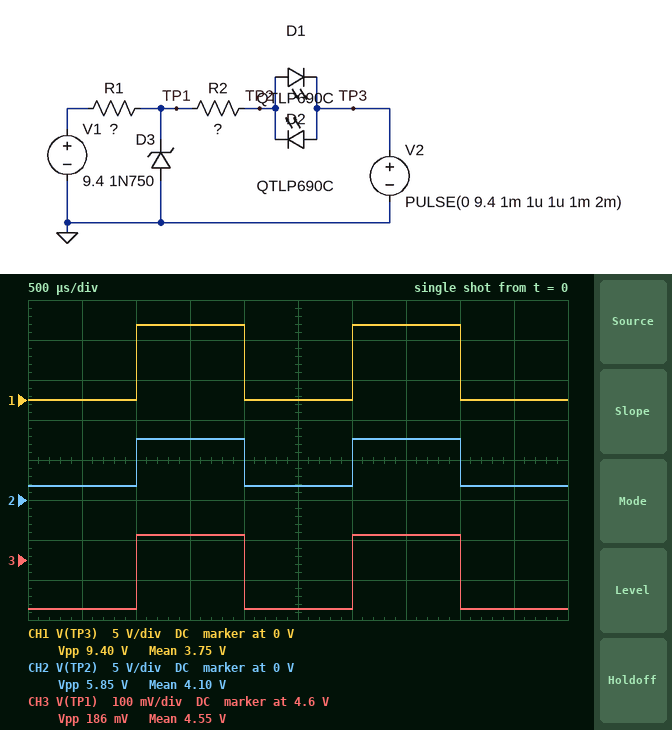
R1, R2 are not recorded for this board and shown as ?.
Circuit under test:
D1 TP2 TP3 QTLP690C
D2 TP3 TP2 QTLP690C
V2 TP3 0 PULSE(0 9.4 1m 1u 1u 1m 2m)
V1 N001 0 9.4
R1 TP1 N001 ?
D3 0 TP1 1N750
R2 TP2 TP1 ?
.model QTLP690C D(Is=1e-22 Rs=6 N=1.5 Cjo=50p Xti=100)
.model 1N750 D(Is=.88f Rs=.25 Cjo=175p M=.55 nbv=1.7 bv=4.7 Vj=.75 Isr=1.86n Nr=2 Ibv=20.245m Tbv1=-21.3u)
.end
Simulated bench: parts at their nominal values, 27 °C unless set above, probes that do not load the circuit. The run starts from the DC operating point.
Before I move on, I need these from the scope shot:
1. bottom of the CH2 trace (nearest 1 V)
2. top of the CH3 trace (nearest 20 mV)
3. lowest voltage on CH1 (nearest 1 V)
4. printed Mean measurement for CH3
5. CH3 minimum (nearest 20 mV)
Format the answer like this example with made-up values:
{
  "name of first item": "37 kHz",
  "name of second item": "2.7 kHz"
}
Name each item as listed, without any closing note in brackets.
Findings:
{
  "bottom of the CH2 trace": "2 V",
  "top of the CH3 trace": "4.66 V",
  "lowest voltage on CH1": "0 V",
  "printed Mean measurement for CH3": "4.55 V",
  "CH3 minimum": "4.48 V"
}
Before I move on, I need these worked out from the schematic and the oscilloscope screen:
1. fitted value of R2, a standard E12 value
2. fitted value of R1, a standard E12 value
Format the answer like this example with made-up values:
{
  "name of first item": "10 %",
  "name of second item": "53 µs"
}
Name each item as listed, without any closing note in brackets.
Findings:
{
  "fitted value of R2, a standard E12 value": "680 Ω",
  "fitted value of R1, a standard E12 value": "1.2 kΩ"
}
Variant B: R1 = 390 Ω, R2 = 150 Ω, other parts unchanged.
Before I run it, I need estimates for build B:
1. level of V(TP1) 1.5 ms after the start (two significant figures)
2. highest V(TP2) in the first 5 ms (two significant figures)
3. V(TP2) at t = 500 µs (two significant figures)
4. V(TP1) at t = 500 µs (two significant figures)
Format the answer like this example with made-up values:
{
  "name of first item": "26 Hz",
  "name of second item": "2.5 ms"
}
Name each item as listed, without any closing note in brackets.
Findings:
{
  "level of V(TP1) 1.5 ms after the start": "4.7 V",
  "highest V(TP2) in the first 5 ms": "7.5 V",
  "V(TP2) at t = 500 µs": "1.9 V",
  "V(TP1) at t = 500 µs": "4.0 V"
}
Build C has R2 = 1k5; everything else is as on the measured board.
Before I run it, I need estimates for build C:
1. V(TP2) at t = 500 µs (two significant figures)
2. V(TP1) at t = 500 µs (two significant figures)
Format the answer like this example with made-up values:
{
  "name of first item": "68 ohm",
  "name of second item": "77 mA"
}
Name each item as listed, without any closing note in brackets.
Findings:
{
  "V(TP2) at t = 500 µs": "1.7 V",
  "V(TP1) at t = 500 µs": "4.6 V"
}
